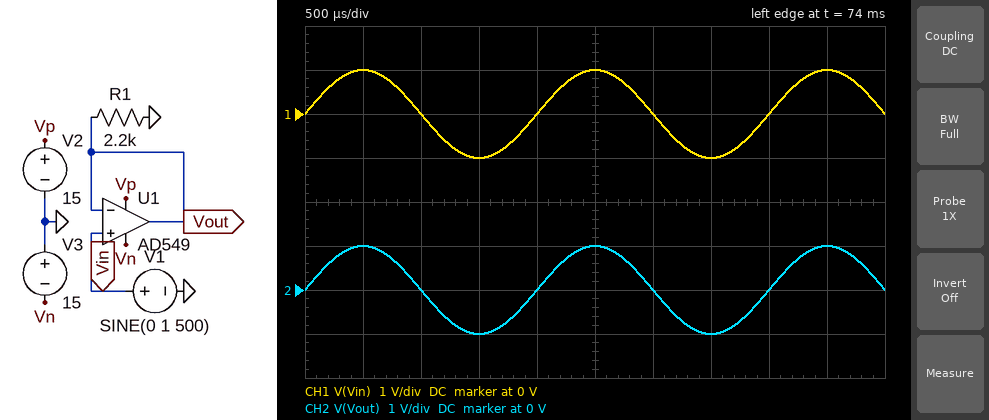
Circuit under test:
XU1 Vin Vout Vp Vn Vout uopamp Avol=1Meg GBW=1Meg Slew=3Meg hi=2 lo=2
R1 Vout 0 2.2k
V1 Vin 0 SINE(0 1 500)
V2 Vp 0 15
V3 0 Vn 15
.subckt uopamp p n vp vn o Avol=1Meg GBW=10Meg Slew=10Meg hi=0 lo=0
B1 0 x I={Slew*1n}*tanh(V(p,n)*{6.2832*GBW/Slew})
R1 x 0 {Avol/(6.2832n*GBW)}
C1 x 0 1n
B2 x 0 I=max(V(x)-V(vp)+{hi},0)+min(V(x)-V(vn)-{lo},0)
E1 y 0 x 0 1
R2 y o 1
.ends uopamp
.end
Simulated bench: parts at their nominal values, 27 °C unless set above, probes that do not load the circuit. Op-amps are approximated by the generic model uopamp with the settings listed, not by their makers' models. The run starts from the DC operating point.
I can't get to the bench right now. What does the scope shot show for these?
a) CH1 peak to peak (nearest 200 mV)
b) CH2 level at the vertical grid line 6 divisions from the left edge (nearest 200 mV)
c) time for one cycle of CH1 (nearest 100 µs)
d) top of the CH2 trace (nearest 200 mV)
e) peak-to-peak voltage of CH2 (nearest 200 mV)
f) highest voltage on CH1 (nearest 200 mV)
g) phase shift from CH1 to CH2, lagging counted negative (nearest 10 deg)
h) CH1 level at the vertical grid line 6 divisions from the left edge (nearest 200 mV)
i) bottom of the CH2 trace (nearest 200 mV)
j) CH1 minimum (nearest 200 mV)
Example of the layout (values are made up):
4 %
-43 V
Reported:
2.0 V
0 V
2.0 ms
1.0 V
2.0 V
1.0 V
0 deg
0 V
-1.0 V
-1.0 V
